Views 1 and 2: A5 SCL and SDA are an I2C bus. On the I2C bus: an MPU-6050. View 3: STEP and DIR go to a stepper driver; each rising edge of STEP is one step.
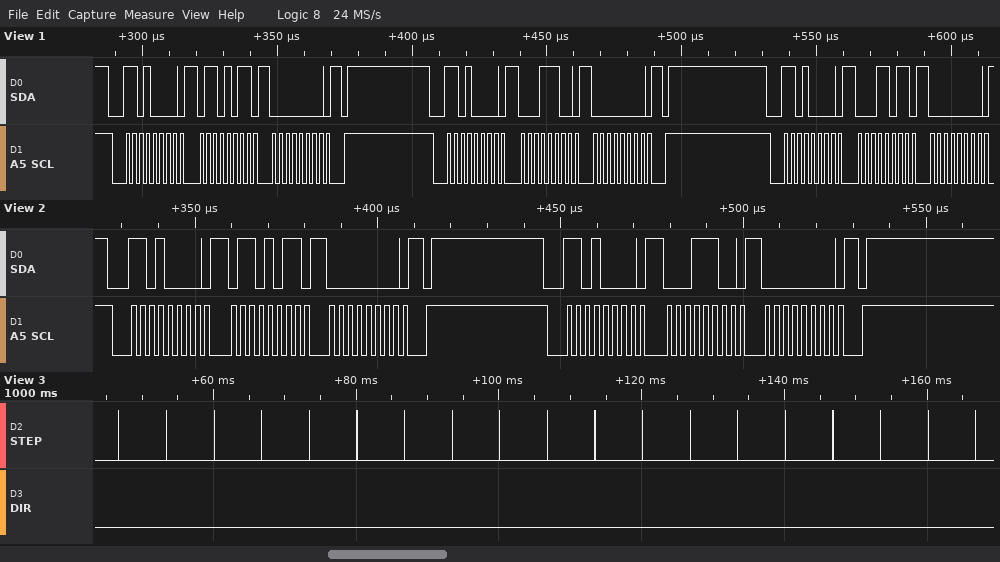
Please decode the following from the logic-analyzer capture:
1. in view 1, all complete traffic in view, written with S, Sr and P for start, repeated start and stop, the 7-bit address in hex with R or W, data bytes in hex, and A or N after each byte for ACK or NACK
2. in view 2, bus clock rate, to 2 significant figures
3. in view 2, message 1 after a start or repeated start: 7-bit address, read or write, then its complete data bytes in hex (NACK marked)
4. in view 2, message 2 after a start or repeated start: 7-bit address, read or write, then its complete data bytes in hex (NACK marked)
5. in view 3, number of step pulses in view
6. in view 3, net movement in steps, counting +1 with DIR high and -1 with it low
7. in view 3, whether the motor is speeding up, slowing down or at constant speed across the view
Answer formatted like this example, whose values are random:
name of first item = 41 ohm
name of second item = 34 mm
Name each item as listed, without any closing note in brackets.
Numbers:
in view 1, all complete traffic in view, written with S, Sr and P for start, repeated start and stop, the 7-bit address in hex with R or W, data bytes in hex, and A or N after each byte for ACK or NACK = S 68W A 6B A 00 A P S 68W A 1C A 00 A P S 68W A 1B A 00 A
in view 2, bus clock rate, to 2 significant figures = 400 kHz
in view 2, message 1 after a start or repeated start: 7-bit address, read or write, then its complete data bytes in hex = 0x68 write: 6B 00
in view 2, message 2 after a start or repeated start: 7-bit address, read or write, then its complete data bytes in hex = 0x68 write: 1C 00
in view 3, number of step pulses in view = 19
in view 3, net movement in steps, counting +1 with DIR high and -1 with it low = -19
in view 3, whether the motor is speeding up, slowing down or at constant speed across the view = constant speed
